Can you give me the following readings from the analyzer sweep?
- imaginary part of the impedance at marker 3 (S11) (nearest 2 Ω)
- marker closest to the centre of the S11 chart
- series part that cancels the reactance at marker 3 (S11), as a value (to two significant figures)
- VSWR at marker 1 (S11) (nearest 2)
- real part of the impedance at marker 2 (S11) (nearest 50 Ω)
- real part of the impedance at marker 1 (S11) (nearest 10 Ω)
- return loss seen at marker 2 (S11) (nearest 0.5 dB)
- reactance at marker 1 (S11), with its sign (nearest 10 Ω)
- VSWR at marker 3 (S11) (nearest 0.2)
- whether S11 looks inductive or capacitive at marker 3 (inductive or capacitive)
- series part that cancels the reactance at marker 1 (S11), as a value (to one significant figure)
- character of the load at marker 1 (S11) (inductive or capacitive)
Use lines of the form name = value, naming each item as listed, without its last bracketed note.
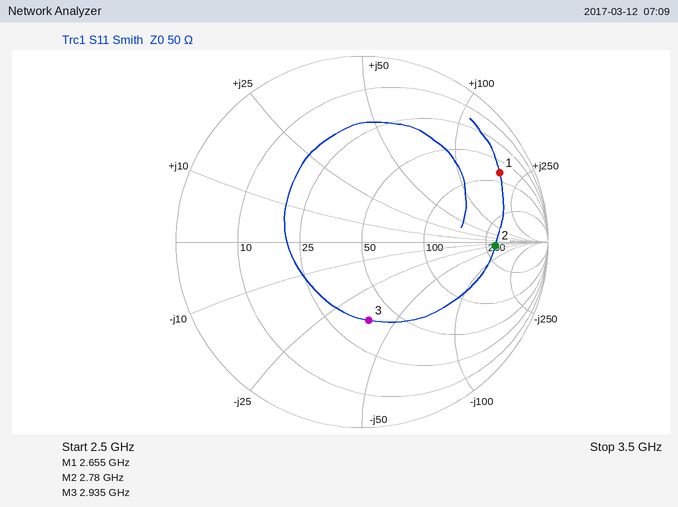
imaginary part of the impedance at marker 3 (S11) = -38 Ω
marker closest to the centre of the S11 chart = marker 3
series part that cancels the reactance at marker 3 (S11), as a value = 2.1 nH
VSWR at marker 1 (S11) = 10
real part of the impedance at marker 2 (S11) = 300 Ω
real part of the impedance at marker 1 (S11) = 80 Ω
return loss seen at marker 2 (S11) = 3.0 dB
reactance at marker 1 (S11), with its sign = +180 Ω
VSWR at marker 3 (S11) = 2.4
whether S11 looks inductive or capacitive at marker 3 = capacitive
series part that cancels the reactance at marker 1 (S11), as a value = 300 fF
character of the load at marker 1 (S11) = inductive
